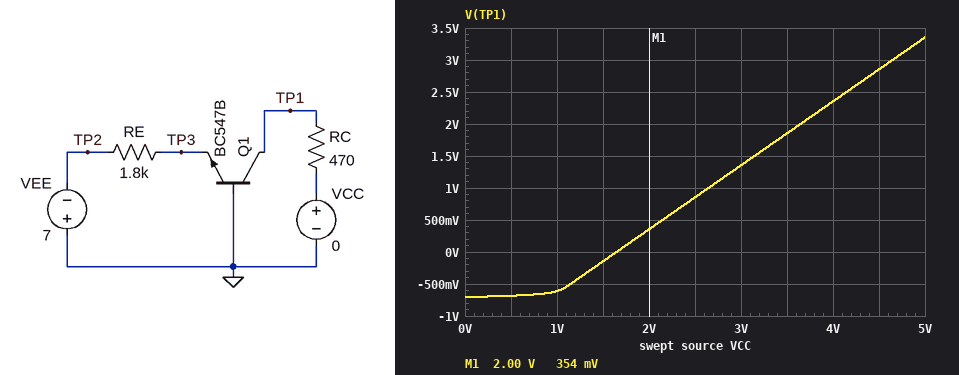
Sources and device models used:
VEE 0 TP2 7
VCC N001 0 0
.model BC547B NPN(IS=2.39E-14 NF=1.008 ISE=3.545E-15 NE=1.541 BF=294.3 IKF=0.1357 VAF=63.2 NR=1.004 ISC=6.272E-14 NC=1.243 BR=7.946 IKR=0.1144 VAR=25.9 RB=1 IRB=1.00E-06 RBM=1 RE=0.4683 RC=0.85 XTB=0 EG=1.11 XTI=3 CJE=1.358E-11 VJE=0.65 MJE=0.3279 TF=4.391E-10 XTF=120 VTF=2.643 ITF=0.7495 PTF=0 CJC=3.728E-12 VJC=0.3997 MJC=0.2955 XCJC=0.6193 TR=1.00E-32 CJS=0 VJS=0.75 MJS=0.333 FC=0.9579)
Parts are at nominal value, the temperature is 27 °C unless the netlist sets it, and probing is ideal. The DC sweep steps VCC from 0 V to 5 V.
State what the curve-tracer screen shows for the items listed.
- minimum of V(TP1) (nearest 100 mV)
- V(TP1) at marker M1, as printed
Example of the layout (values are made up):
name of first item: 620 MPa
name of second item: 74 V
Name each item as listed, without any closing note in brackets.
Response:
minimum of V(TP1): -700 mV
V(TP1) at marker M1, as printed: 354 mV
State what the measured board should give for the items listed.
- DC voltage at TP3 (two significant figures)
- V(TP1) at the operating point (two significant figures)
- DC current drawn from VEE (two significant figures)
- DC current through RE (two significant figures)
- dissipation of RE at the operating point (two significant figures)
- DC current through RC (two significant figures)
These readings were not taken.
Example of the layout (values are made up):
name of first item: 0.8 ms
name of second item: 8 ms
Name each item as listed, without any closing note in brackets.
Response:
DC voltage at TP3: -720 mV
V(TP1) at the operating point: -700 mV
DC current drawn from VEE: 3.5 mA
DC current through RE: 3.5 mA
dissipation of RE at the operating point: 22 mW
DC current through RC: 1.5 mA
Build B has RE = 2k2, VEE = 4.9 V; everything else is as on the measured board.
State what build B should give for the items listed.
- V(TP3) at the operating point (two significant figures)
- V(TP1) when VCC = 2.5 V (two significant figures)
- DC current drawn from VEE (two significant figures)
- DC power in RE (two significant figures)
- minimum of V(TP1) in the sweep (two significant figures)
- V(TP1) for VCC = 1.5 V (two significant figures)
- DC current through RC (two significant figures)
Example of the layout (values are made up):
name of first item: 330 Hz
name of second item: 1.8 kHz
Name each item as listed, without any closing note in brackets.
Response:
V(TP3) at the operating point: -680 mV
V(TP1) when VCC = 2.5 V: 1.6 V
DC current drawn from VEE: 1.9 mA
DC power in RE: 8.1 mW
minimum of V(TP1) in the sweep: -670 mV
V(TP1) for VCC = 1.5 V: 600 mV
DC current through RC: 1.4 mA
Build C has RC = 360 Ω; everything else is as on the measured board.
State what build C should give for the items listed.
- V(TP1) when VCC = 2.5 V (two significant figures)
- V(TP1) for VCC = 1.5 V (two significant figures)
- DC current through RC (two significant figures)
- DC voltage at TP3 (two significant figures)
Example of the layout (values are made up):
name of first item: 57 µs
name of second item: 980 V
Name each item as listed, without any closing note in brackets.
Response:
V(TP1) when VCC = 2.5 V: 1.2 V
V(TP1) for VCC = 1.5 V: 240 mV
DC current through RC: 1.9 mA
DC voltage at TP3: -710 mV
